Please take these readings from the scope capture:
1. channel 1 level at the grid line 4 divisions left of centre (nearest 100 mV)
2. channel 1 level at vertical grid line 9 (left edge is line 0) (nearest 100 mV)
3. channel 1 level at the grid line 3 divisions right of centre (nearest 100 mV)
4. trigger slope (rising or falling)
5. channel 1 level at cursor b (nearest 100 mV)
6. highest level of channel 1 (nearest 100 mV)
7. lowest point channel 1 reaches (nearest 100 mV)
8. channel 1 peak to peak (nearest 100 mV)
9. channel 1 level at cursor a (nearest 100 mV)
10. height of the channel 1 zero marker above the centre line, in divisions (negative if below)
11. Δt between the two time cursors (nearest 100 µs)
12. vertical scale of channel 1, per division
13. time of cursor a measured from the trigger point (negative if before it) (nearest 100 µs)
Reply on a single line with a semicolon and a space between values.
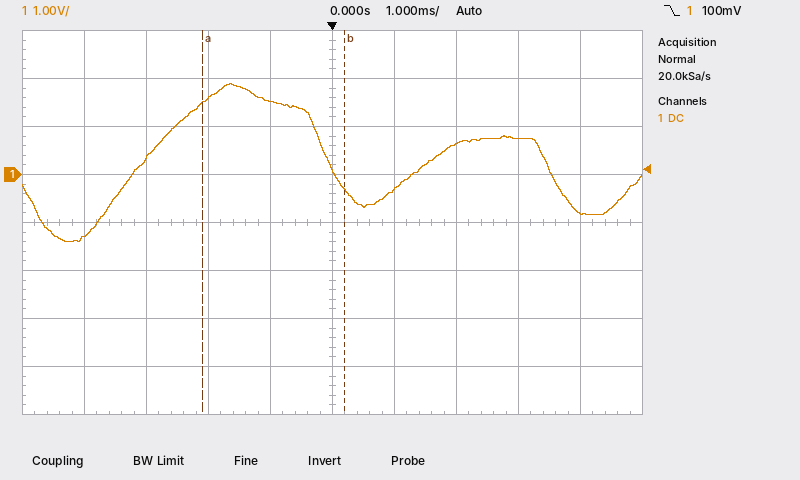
-1.3 V; -800 mV; 800 mV; falling; -300 mV; 1.9 V; -1.4 V; 3.3 V; 1.5 V; +1.0 div; 2.3 ms; 1 V; -2.1 ms
